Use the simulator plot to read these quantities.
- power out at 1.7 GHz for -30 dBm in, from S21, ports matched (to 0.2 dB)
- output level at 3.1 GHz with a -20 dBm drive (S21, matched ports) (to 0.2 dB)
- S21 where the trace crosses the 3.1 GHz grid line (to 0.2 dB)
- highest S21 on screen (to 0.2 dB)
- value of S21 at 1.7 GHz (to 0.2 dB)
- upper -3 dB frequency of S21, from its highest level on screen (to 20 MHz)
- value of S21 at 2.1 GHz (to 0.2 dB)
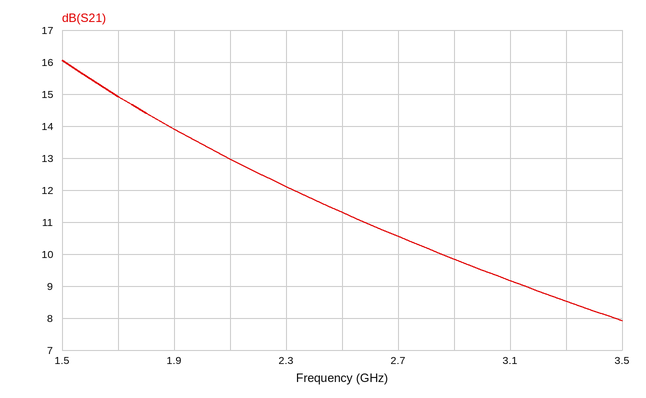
-15.0 dBm
-10.8 dBm
9.2 dB
16.0 dB
15.0 dB
2.08 GHz
13.0 dB
